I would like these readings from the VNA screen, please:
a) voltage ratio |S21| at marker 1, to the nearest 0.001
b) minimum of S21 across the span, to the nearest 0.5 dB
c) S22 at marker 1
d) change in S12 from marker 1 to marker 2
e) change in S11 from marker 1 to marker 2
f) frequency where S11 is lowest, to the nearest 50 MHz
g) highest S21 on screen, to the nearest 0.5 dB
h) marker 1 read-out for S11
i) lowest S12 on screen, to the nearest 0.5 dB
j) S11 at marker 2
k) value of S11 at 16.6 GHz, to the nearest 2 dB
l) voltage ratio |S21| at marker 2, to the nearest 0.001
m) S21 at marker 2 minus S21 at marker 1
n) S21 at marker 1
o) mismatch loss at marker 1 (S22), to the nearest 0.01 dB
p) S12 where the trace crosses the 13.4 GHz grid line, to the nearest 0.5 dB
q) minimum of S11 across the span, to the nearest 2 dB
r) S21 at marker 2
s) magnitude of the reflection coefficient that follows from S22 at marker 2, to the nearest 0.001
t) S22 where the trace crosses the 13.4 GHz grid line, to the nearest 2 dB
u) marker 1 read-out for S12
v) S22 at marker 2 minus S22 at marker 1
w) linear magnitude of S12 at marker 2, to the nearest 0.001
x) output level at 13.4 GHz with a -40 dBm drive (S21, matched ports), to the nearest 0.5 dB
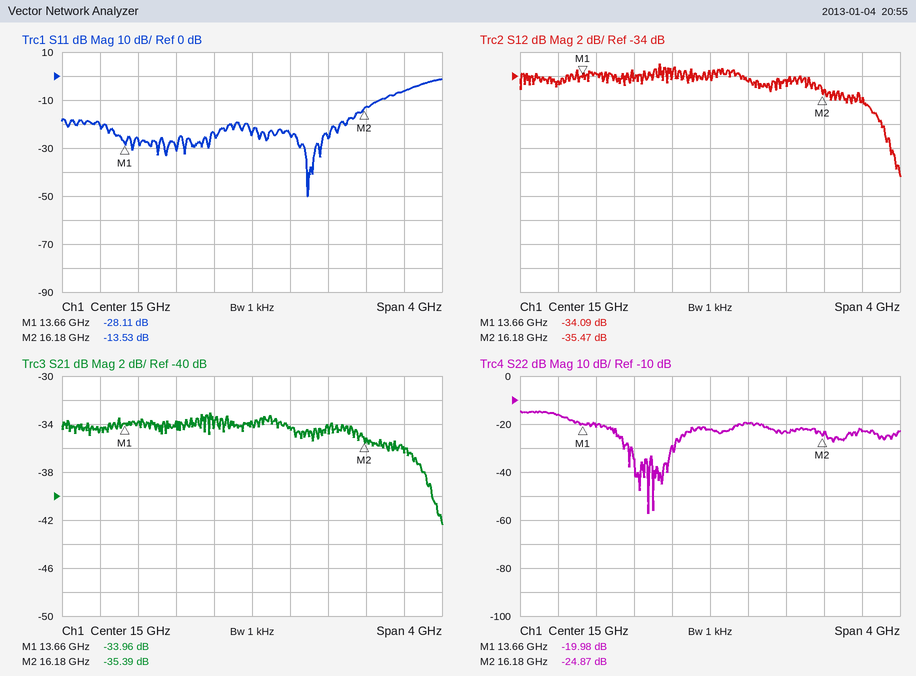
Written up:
0.020
-42.5 dB
-19.98 dB
-1.38 dB
14.58 dB
15.60 GHz
-33.0 dB
-28.11 dB
-42.5 dB
-13.53 dB
-6 dB
0.017
-1.43 dB
-33.96 dB
0.04 dB
-34.5 dB
-50 dB
-35.39 dB
0.057
-16 dB
-34.09 dB
-4.89 dB
0.017
-74.5 dBm
